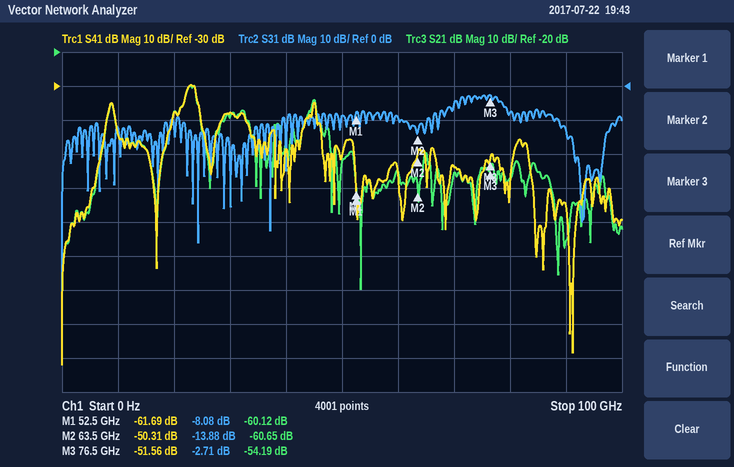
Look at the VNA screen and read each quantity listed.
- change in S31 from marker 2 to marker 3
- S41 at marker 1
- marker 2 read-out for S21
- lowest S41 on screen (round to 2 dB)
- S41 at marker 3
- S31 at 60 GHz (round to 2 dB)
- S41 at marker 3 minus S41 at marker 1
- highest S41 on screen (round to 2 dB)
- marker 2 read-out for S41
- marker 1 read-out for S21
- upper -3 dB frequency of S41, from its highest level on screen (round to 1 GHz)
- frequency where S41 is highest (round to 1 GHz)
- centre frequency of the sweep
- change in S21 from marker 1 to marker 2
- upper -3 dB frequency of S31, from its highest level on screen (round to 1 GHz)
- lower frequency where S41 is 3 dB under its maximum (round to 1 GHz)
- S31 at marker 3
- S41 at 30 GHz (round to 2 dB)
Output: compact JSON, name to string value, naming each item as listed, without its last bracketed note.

{"change in S31 from marker 2 to marker 3": "11.17 dB", "S41 at marker 1": "-61.69 dB", "marker 2 read-out for S21": "-60.65 dB", "lowest S41 on screen": "-112 dB", "S41 at marker 3": "-51.56 dB", "S31 at 60 GHz": "-10 dB", "S41 at marker 3 minus S41 at marker 1": "10.13 dB", "highest S41 on screen": "-30 dB", "marker 2 read-out for S41": "-50.31 dB", "marker 1 read-out for S21": "-60.12 dB", "upper -3 dB frequency of S41, from its highest level on screen": "24 GHz", "frequency where S41 is highest": "23 GHz", "centre frequency of the sweep": "50 GHz", "change in S21 from marker 1 to marker 2": "-0.53 dB", "upper -3 dB frequency of S31, from its highest level on screen": "79 GHz", "lower frequency where S41 is 3 dB under its maximum": "22 GHz", "S31 at marker 3": "-2.71 dB", "S41 at 30 GHz": "-38 dB"}
